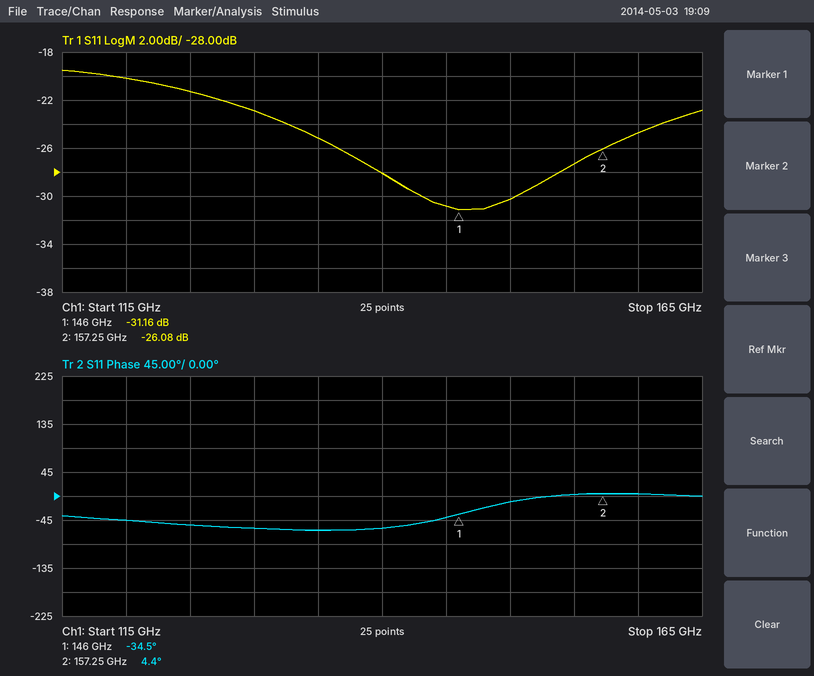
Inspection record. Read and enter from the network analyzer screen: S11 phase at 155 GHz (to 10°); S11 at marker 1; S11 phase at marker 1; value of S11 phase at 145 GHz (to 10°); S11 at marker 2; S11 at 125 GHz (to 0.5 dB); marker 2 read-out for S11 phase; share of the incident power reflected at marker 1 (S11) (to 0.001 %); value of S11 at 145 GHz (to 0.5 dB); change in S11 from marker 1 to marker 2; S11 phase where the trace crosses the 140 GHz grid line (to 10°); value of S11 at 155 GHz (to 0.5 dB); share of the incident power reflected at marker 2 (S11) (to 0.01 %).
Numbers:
0°
-31.16 dB
-34.5°
-40°
-26.08 dB
-21.5 dB
4.4°
0.077 %
-31.0 dB
5.08 dB
-60°
-27.5 dB
0.25 %
